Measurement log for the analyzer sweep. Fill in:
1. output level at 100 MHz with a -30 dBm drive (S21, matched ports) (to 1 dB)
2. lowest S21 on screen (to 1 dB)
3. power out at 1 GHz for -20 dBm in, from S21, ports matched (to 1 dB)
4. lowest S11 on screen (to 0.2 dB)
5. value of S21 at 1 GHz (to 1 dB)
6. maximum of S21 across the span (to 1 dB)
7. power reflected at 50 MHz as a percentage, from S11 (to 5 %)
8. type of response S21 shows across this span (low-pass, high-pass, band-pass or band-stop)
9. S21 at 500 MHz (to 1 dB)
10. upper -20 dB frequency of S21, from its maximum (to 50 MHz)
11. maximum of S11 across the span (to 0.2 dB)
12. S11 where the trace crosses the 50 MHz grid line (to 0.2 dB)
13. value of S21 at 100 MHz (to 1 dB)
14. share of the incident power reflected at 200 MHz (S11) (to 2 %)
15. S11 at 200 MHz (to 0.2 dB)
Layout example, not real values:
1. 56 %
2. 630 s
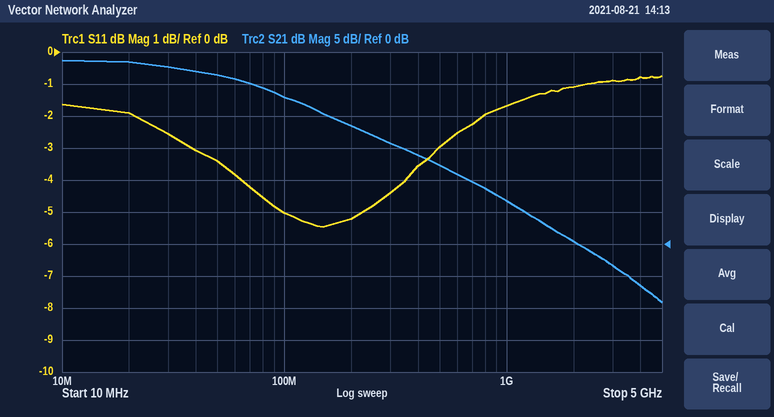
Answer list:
1. -7 dBm
2. -9 dB
3. -13 dBm
4. -5.4 dB
5. 7 dB
6. 29 dB
7. 45 %
8. low-pass
9. 12 dB
10. 800 MHz
11. -0.8 dB
12. -3.4 dB
13. 23 dB
14. 30 %
15. -5.2 dB
